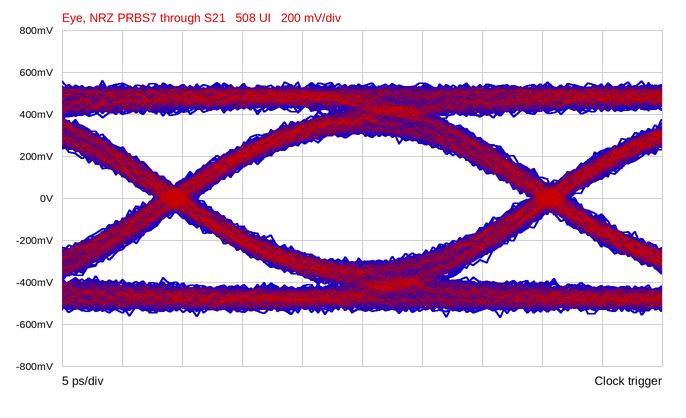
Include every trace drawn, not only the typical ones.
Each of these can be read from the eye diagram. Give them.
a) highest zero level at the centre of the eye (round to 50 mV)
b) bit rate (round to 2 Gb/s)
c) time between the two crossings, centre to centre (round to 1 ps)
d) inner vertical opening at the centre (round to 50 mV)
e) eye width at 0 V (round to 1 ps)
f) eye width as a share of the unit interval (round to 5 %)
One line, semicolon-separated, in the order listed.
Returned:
-300 mV; 32 Gb/s; 31 ps; 600 mV; 28 ps; 90 %
